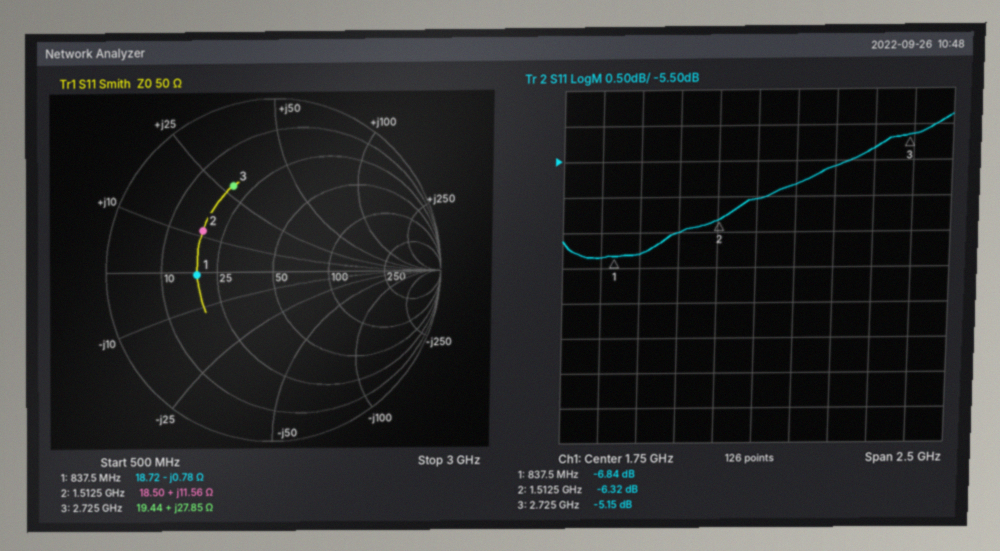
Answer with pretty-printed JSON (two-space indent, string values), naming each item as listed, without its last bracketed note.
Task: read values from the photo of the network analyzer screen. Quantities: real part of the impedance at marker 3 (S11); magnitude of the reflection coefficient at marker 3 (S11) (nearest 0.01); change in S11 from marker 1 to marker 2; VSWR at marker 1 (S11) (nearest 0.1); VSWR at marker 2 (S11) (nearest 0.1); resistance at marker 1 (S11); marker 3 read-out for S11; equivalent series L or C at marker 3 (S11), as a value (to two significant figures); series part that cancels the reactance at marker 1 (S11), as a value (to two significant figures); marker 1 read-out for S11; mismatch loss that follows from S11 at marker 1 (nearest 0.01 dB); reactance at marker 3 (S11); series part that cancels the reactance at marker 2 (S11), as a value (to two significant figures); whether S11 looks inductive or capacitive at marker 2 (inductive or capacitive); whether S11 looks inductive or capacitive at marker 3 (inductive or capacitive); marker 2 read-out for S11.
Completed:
{
  "real part of the impedance at marker 3": "19.44 Ω",
  "magnitude of the reflection coefficient at marker 3 (S11)": "0.55",
  "change in S11 from marker 1 to marker 2": "0.52 dB",
  "VSWR at marker 1 (S11)": "2.7",
  "VSWR at marker 2 (S11)": "2.9",
  "resistance at marker 1": "18.72 Ω",
  "marker 3 read-out for S11": "-5.15 dB",
  "equivalent series L or C at marker 3 (S11), as a value": "1.6 nH",
  "series part that cancels the reactance at marker 1 (S11), as a value": "150 pH",
  "marker 1 read-out for S11": "-6.84 dB",
  "mismatch loss that follows from S11 at marker 1": "1.01 dB",
  "reactance at marker 3": "+27.85 Ω",
  "series part that cancels the reactance at marker 2 (S11), as a value": "9.1 pF",
  "whether S11 looks inductive or capacitive at marker 2": "inductive",
  "whether S11 looks inductive or capacitive at marker 3": "inductive",
  "marker 2 read-out for S11": "-6.32 dB"
}
